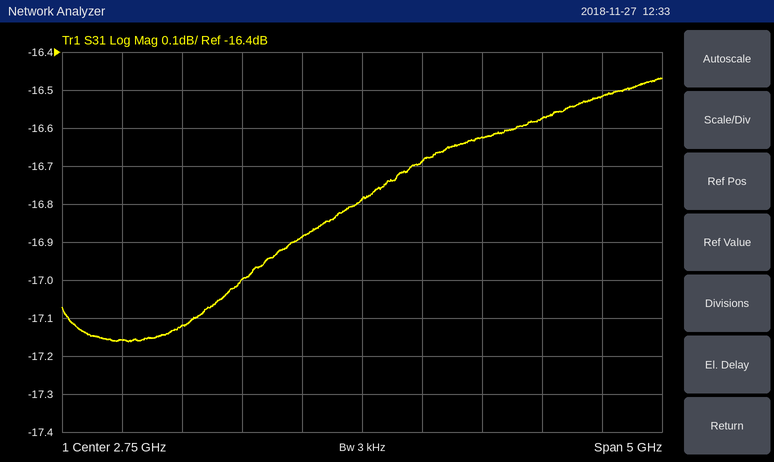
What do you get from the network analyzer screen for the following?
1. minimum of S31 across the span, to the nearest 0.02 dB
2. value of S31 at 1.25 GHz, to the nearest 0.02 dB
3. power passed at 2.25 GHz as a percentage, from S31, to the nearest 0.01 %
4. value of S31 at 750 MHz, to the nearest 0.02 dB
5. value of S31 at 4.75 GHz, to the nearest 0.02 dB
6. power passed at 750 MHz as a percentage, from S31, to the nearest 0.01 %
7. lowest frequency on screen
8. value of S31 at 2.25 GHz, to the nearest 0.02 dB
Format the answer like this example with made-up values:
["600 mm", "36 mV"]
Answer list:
["-17.16 dB", "-17.12 dB", "2.05 %", "-17.16 dB", "-16.52 dB", "1.92 %", "250 MHz", "-16.88 dB"]
